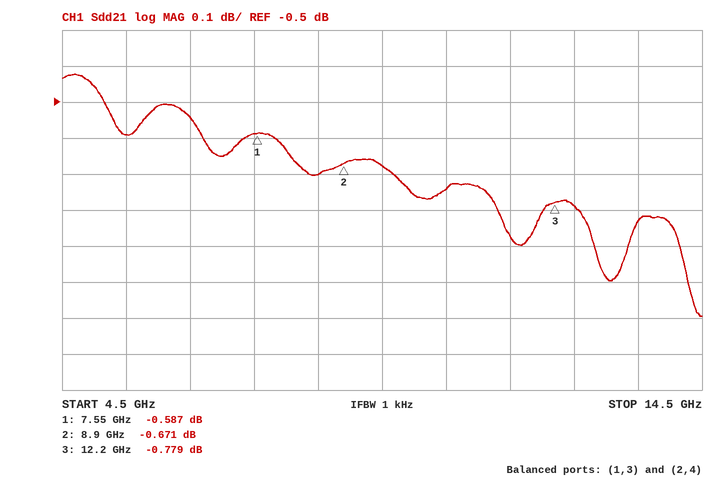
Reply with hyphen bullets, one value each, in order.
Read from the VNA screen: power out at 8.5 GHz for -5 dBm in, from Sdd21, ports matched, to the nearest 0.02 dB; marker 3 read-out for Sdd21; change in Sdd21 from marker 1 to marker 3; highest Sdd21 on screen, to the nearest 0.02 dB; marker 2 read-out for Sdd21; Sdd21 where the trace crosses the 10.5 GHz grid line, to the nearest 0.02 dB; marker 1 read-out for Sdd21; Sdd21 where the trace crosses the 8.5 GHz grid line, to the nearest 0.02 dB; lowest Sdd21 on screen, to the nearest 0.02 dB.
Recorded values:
- -5.70 dBm
- -0.779 dB
- -0.192 dB
- -0.42 dB
- -0.671 dB
- -0.74 dB
- -0.587 dB
- -0.70 dB
- -1.10 dB
